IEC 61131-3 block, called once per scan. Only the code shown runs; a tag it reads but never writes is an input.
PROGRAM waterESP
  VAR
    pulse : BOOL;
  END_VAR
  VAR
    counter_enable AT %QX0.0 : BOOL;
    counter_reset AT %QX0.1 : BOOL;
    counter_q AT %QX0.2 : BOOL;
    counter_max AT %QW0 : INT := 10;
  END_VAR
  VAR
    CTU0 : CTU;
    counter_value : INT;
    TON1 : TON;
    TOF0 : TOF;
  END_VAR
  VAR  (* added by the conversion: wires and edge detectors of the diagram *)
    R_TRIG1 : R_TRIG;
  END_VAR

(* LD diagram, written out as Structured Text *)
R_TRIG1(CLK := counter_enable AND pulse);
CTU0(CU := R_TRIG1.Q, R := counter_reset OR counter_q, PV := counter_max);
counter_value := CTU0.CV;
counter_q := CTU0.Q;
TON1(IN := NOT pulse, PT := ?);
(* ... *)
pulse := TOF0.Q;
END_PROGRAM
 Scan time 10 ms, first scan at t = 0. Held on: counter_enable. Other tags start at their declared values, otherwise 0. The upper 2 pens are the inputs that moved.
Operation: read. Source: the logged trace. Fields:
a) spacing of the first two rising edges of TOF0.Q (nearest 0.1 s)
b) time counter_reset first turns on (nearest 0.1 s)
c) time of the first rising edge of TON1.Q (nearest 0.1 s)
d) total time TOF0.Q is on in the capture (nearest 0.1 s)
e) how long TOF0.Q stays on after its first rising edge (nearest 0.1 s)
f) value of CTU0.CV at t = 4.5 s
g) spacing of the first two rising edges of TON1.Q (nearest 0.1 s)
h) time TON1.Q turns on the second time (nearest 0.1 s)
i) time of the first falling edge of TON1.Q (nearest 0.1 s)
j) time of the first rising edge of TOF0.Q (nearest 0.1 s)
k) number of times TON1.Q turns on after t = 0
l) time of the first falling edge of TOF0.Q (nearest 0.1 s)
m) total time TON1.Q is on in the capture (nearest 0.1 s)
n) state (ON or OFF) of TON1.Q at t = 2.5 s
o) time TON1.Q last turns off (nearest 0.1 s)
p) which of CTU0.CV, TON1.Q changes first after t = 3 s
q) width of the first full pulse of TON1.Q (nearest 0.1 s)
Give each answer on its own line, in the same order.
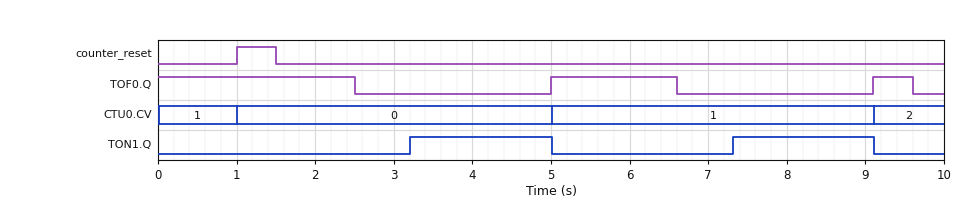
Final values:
4.1 s
1.0 s
3.2 s
4.6 s
1.6 s
0
4.1 s
7.3 s
5.0 s
5.0 s
2
2.5 s
3.6 s
OFF
9.1 s
TON1.Q
1.8 s
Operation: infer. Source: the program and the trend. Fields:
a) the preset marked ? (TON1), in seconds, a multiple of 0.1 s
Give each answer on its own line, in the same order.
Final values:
0.7 s
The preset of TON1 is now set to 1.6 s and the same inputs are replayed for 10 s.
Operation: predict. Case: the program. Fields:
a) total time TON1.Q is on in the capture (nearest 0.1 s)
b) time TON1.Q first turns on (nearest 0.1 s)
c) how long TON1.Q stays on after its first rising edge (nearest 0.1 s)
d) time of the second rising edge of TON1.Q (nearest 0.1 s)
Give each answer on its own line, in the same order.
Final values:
1.8 s
4.1 s
0.9 s
8.2 s
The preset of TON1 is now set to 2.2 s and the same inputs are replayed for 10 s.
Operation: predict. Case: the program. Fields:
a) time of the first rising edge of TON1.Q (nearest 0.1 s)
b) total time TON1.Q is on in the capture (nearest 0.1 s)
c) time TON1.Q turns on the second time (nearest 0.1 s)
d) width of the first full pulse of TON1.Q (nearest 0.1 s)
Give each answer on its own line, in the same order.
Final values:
4.7 s
0.6 s
8.8 s
0.3 s
